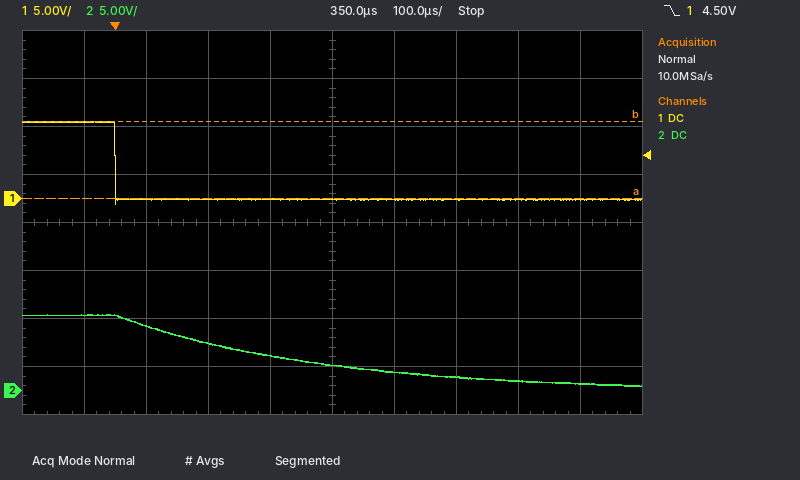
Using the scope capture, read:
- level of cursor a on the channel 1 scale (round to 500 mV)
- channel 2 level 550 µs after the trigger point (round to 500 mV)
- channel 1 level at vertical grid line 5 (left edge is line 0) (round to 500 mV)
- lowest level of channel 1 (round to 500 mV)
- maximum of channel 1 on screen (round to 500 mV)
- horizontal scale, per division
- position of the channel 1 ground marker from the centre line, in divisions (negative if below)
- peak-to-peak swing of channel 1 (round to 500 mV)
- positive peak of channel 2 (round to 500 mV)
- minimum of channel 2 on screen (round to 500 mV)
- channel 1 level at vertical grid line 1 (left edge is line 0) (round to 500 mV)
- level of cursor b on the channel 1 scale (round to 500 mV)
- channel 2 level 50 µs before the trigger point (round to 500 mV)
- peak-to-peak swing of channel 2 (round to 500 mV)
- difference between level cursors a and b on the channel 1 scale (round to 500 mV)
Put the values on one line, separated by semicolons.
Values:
0.0 V; 1.5 V; 0.0 V; -500 mV; 8.0 V; 100 µs; +0.5 div; 8.5 V; 8.0 V; 500 mV; 8.0 V; 8.0 V; 8.0 V; 7.5 V; 8.0 V
